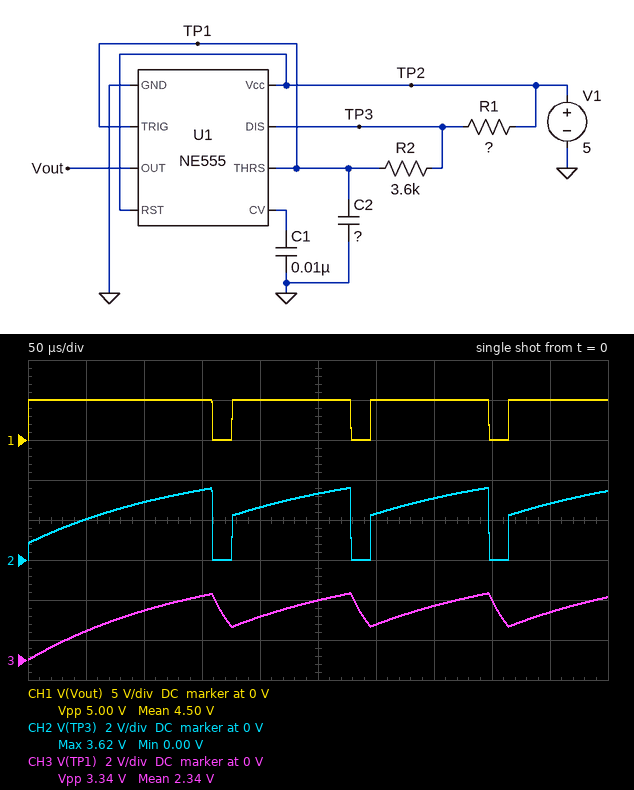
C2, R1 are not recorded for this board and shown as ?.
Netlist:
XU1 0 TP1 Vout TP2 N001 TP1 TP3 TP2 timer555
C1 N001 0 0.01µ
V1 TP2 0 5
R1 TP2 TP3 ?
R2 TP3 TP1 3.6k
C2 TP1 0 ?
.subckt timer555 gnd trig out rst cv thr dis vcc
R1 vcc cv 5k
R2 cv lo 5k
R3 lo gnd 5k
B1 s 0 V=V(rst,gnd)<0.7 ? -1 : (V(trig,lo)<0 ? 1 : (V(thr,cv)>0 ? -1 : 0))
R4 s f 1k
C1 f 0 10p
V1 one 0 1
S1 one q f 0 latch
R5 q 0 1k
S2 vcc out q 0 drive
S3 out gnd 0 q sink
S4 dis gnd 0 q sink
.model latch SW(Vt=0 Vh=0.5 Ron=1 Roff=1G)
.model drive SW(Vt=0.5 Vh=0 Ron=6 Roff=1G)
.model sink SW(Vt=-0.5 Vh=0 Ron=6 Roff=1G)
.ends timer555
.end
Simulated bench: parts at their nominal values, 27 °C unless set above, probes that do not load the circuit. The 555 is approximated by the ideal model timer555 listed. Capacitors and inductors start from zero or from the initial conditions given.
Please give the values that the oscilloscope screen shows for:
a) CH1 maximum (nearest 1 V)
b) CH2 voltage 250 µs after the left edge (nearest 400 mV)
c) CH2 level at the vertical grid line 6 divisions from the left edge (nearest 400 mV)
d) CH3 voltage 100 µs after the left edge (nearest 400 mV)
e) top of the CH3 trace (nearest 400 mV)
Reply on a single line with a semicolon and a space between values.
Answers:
5 V; 3.2 V; 2.4 V; 2.4 V; 3.2 V
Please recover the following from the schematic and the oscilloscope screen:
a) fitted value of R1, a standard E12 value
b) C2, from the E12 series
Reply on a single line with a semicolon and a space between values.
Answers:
18 kΩ; 6.8 nF
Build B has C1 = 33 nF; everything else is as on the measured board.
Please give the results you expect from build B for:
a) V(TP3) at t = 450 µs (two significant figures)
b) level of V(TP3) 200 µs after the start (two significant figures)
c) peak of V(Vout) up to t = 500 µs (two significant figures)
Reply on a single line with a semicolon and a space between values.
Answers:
3.5 V; 2.9 V; 5.0 V
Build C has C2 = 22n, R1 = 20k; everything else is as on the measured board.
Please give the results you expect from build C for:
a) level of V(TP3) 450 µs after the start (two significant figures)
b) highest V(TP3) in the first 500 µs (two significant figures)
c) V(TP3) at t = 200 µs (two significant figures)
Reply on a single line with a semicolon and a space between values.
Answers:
3.2 V; 3.4 V; 2.1 V
